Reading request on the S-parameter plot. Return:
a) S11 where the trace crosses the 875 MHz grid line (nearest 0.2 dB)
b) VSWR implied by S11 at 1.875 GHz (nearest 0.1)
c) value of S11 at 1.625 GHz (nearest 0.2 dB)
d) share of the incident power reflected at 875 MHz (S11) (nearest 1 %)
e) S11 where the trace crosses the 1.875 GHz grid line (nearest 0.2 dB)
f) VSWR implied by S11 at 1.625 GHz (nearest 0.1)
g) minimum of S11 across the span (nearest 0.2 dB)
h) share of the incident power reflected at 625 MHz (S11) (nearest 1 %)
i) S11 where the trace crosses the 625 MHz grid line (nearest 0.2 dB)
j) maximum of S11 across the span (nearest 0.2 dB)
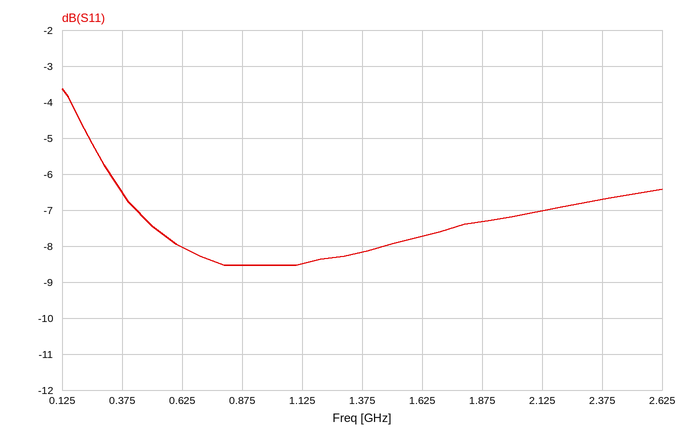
-8.6 dB
2.5
-7.8 dB
14 %
-7.4 dB
2.4
-8.6 dB
16 %
-8.0 dB
-3.6 dB
